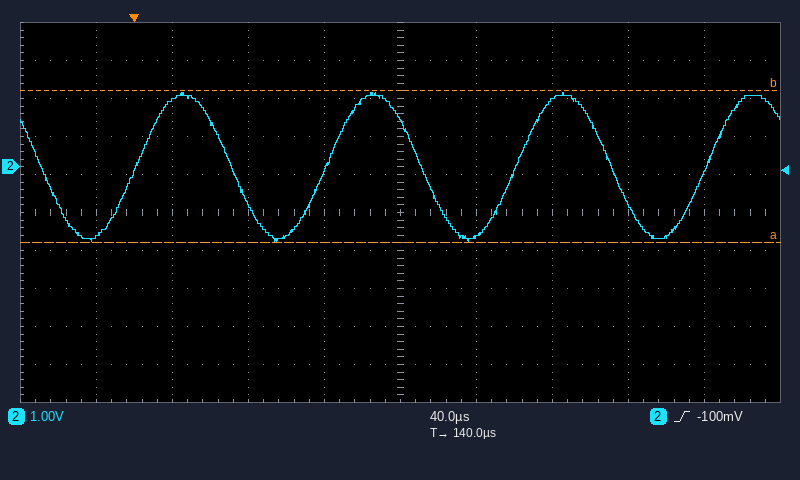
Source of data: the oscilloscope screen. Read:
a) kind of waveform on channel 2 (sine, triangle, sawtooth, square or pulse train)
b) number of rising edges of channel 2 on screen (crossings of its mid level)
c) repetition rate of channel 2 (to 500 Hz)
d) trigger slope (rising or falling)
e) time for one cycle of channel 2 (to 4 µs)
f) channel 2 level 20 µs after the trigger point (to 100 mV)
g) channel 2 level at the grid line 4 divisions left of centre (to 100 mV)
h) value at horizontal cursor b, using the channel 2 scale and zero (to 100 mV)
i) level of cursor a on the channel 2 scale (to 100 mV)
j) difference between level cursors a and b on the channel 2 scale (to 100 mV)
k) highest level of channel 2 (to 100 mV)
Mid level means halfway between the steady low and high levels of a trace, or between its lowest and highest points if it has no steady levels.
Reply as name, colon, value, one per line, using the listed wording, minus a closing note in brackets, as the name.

kind of waveform on channel 2: sine
number of rising edges of channel 2 on screen: 4
repetition rate of channel 2: 10.0 kHz
trigger slope: rising
time for one cycle of channel 2: 100 µs
channel 2 level 20 µs after the trigger point: 1.8 V
channel 2 level at the grid line 4 divisions left of centre: -1.8 V
value at horizontal cursor b, using the channel 2 scale and zero: 2.0 V
level of cursor a on the channel 2 scale: -2.0 V
difference between level cursors a and b on the channel 2 scale: 4.0 V
highest level of channel 2: 2.0 V
